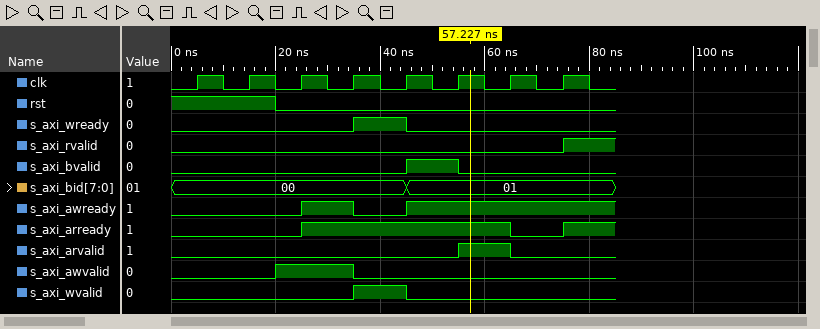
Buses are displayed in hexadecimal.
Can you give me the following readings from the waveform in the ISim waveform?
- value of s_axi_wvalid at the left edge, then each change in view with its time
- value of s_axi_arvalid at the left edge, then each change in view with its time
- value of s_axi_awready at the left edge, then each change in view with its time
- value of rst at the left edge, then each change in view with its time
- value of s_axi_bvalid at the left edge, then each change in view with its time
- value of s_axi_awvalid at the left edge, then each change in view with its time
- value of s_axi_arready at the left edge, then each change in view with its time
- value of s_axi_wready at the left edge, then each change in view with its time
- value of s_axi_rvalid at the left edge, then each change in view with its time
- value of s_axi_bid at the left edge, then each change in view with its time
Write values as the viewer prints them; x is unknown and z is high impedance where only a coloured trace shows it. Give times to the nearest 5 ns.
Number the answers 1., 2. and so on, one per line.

1. 0, 1 at 35 ns, 0 at 45 ns
2. 0, 1 at 55 ns, 0 at 65 ns
3. 0, 1 at 25 ns, 0 at 35 ns, 1 at 45 ns
4. 1, 0 at 20 ns
5. 0, 1 at 45 ns, 0 at 55 ns
6. 0, 1 at 20 ns, 0 at 35 ns
7. 0, 1 at 25 ns, 0 at 65 ns, 1 at 75 ns
8. 0, 1 at 35 ns, 0 at 45 ns
9. 0, 1 at 75 ns
10. 00, 01 at 45 ns
